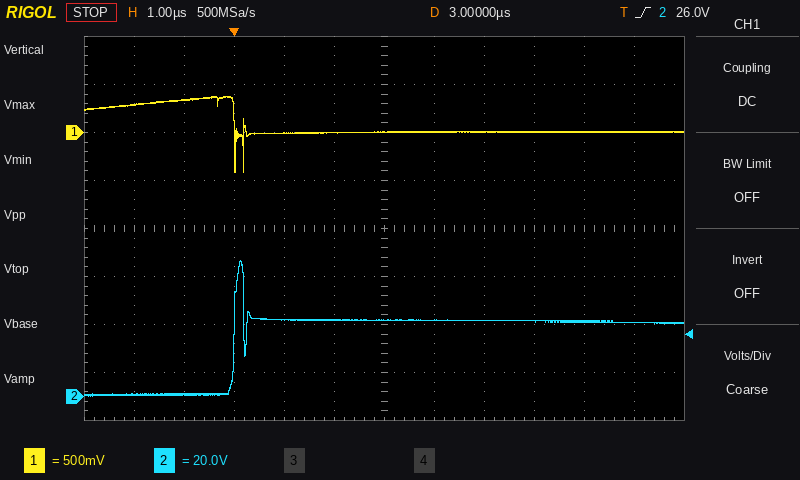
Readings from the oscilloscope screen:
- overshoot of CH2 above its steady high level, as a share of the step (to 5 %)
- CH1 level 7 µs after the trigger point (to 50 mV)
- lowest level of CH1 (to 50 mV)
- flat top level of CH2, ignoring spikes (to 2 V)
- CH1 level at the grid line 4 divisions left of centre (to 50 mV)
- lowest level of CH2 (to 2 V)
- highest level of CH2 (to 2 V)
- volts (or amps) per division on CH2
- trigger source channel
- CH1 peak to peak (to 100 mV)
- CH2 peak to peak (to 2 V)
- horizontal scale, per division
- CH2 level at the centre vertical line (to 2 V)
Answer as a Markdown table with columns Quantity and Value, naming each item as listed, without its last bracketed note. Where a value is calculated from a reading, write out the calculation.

| Quantity | Value |
|---|---|
| overshoot of CH2 above its steady high level, as a share of the step | 80 % |
| CH1 level 7 µs after the trigger point | 0 mV |
| lowest level of CH1 | -400 mV |
| flat top level of CH2, ignoring spikes | 32 V |
| CH1 level at the grid line 4 divisions left of centre | 350 mV |
| lowest level of CH2 | 0 V |
| highest level of CH2 | 56 V |
| volts (or amps) per division on CH2 | 20 V |
| trigger source channel | CH2 |
| CH1 peak to peak | 800 mV |
| CH2 peak to peak | 56 V − (0 V) = 56 V |
| horizontal scale, per division | 1 µs |
| CH2 level at the centre vertical line | 32 V |
